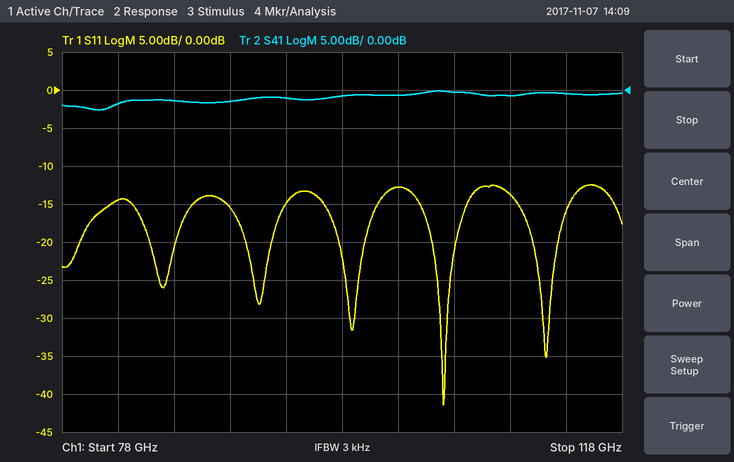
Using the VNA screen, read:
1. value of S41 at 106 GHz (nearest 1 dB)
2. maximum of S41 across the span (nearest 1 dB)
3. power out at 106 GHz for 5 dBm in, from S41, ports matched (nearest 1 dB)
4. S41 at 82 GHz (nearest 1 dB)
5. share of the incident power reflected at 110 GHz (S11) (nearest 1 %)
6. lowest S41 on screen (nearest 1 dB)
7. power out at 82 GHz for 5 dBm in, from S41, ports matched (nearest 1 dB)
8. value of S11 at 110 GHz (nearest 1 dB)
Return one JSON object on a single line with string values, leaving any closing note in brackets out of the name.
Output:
{"value of S41 at 106 GHz": "0 dB", "maximum of S41 across the span": "0 dB", "power out at 106 GHz for 5 dBm in, from S41, ports matched": "5 dBm", "S41 at 82 GHz": "-2 dB", "share of the incident power reflected at 110 GHz (S11)": "4 %", "lowest S41 on screen": "-3 dB", "power out at 82 GHz for 5 dBm in, from S41, ports matched": "3 dBm", "value of S11 at 110 GHz": "-14 dB"}
